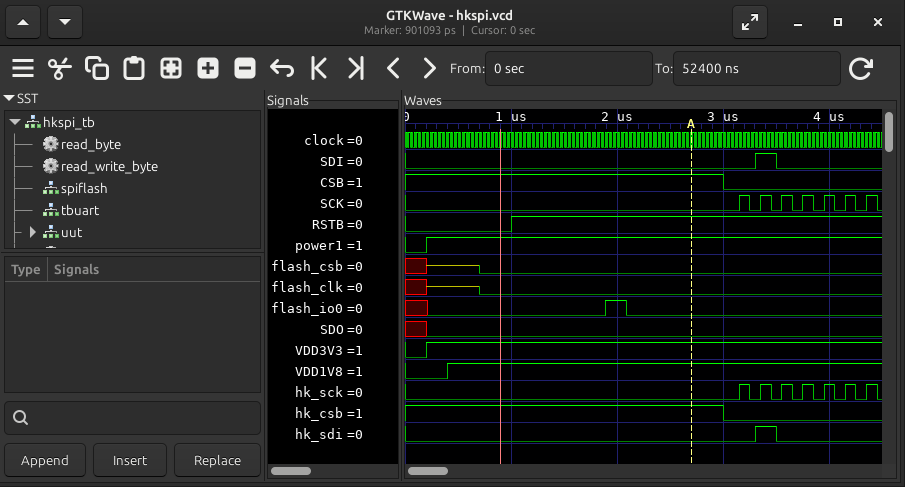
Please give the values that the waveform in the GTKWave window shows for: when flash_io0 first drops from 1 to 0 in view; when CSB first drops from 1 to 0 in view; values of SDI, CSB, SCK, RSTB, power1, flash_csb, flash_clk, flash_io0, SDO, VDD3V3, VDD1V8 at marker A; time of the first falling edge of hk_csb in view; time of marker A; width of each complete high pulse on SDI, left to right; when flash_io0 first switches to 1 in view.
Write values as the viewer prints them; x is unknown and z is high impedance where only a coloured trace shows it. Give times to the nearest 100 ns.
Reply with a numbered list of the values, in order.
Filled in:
1. 2100 ns
2. 3000 ns
3. SDI=0, CSB=1, SCK=0, RSTB=1, power1=1, flash_csb=0, flash_clk=0, flash_io0=0, SDO=0, VDD3V3=1, VDD1V8=1
4. 3000 ns
5. 2700 ns
6. 200 ns
7. 1900 ns
